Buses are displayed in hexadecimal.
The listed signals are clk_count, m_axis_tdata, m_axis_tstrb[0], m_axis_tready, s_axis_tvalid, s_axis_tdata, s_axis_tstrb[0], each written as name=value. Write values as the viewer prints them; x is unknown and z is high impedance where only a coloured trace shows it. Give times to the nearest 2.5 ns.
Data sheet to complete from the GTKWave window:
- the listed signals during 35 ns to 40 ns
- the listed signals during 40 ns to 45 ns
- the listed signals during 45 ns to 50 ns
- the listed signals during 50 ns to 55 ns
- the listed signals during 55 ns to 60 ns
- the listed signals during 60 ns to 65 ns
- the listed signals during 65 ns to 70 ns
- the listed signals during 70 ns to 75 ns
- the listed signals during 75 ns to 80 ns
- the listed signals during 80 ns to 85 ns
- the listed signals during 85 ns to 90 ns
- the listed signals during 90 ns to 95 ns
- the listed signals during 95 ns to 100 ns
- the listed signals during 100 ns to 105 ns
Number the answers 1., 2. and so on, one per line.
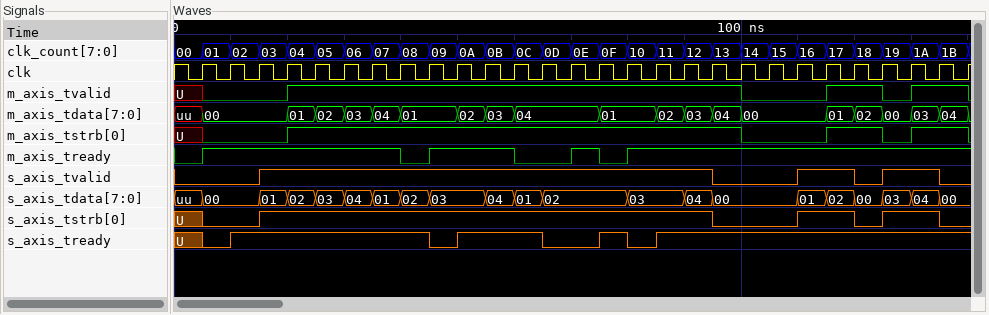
1. clk_count=07, m_axis_tdata=04, m_axis_tstrb[0]=1, m_axis_tready=1, s_axis_tvalid=1, s_axis_tdata=01, s_axis_tstrb[0]=1
2. clk_count=08, m_axis_tdata=01, m_axis_tstrb[0]=1, m_axis_tready=0, s_axis_tvalid=1, s_axis_tdata=02, s_axis_tstrb[0]=1
3. clk_count=09, m_axis_tdata=01, m_axis_tstrb[0]=1, m_axis_tready=1, s_axis_tvalid=1, s_axis_tdata=03, s_axis_tstrb[0]=1
4. clk_count=0A, m_axis_tdata=02, m_axis_tstrb[0]=1, m_axis_tready=1, s_axis_tvalid=1, s_axis_tdata=03, s_axis_tstrb[0]=1
5. clk_count=0B, m_axis_tdata=03, m_axis_tstrb[0]=1, m_axis_tready=1, s_axis_tvalid=1, s_axis_tdata=04, s_axis_tstrb[0]=1
6. clk_count=0C, m_axis_tdata=04, m_axis_tstrb[0]=1, m_axis_tready=0, s_axis_tvalid=1, s_axis_tdata=01, s_axis_tstrb[0]=1
7. clk_count=0D, m_axis_tdata=04, m_axis_tstrb[0]=1, m_axis_tready=0, s_axis_tvalid=1, s_axis_tdata=02, s_axis_tstrb[0]=1
8. clk_count=0E, m_axis_tdata=04, m_axis_tstrb[0]=1, m_axis_tready=1, s_axis_tvalid=1, s_axis_tdata=02, s_axis_tstrb[0]=1
9. clk_count=0F, m_axis_tdata=01, m_axis_tstrb[0]=1, m_axis_tready=0, s_axis_tvalid=1, s_axis_tdata=02, s_axis_tstrb[0]=1
10. clk_count=10, m_axis_tdata=01, m_axis_tstrb[0]=1, m_axis_tready=1, s_axis_tvalid=1, s_axis_tdata=03, s_axis_tstrb[0]=1
11. clk_count=11, m_axis_tdata=02, m_axis_tstrb[0]=1, m_axis_tready=1, s_axis_tvalid=1, s_axis_tdata=03, s_axis_tstrb[0]=1
12. clk_count=12, m_axis_tdata=03, m_axis_tstrb[0]=1, m_axis_tready=1, s_axis_tvalid=1, s_axis_tdata=04, s_axis_tstrb[0]=1
13. clk_count=13, m_axis_tdata=04, m_axis_tstrb[0]=1, m_axis_tready=1, s_axis_tvalid=0, s_axis_tdata=00, s_axis_tstrb[0]=0
14. clk_count=14, m_axis_tdata=00, m_axis_tstrb[0]=0, m_axis_tready=1, s_axis_tvalid=0, s_axis_tdata=00, s_axis_tstrb[0]=0
